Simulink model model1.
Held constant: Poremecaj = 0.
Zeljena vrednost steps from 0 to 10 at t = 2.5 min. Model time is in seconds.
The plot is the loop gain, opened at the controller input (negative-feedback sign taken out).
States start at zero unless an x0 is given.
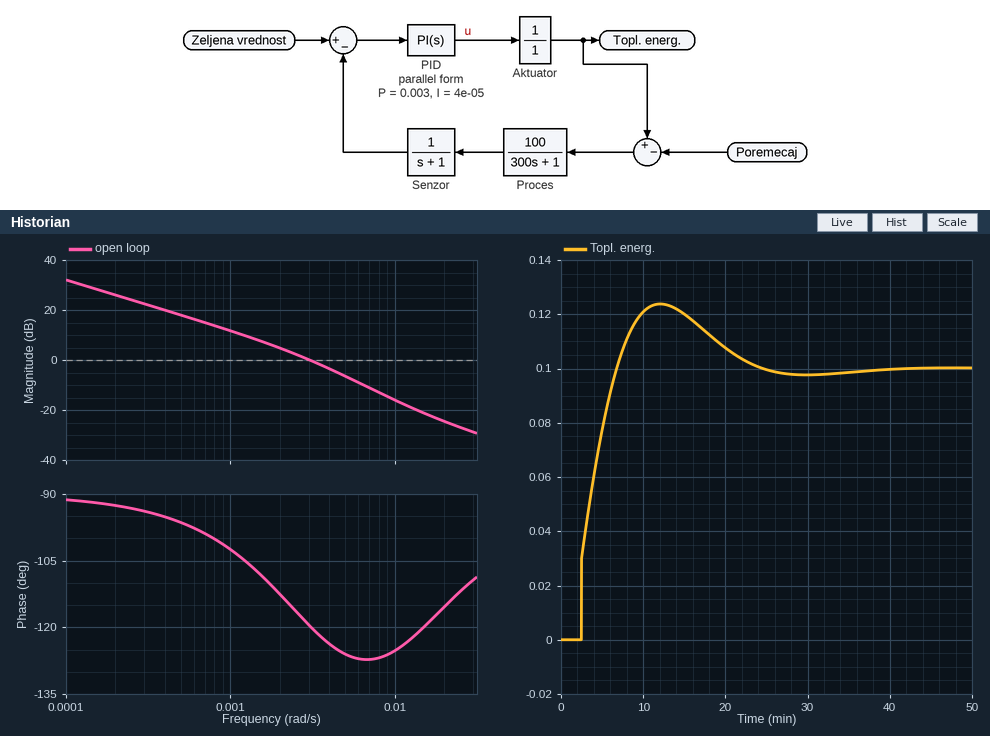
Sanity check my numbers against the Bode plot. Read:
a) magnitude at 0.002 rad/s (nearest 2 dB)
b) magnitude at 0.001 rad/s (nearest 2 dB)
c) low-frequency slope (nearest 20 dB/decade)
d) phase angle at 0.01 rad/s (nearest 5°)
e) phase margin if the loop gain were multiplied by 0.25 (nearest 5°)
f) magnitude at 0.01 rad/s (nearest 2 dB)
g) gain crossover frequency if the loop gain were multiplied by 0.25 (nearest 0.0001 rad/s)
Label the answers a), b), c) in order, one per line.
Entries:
a) 4 dB
b) 12 dB
c) -20 dB/decade
d) -125°
e) 80°
f) -16 dB
g) 0.0010 rad/s
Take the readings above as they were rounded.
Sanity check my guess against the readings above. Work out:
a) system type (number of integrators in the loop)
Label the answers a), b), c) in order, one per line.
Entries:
a) 1
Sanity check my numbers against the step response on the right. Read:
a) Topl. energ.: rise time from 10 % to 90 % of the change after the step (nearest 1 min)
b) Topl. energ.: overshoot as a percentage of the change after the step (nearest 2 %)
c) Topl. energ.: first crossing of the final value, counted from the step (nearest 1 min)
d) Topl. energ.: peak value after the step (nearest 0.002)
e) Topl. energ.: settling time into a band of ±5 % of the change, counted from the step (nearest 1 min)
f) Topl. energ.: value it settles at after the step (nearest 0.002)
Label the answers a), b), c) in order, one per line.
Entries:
a) 3 min
b) 24 %
c) 4 min
d) 0.124
e) 19 min
f) 0.100
